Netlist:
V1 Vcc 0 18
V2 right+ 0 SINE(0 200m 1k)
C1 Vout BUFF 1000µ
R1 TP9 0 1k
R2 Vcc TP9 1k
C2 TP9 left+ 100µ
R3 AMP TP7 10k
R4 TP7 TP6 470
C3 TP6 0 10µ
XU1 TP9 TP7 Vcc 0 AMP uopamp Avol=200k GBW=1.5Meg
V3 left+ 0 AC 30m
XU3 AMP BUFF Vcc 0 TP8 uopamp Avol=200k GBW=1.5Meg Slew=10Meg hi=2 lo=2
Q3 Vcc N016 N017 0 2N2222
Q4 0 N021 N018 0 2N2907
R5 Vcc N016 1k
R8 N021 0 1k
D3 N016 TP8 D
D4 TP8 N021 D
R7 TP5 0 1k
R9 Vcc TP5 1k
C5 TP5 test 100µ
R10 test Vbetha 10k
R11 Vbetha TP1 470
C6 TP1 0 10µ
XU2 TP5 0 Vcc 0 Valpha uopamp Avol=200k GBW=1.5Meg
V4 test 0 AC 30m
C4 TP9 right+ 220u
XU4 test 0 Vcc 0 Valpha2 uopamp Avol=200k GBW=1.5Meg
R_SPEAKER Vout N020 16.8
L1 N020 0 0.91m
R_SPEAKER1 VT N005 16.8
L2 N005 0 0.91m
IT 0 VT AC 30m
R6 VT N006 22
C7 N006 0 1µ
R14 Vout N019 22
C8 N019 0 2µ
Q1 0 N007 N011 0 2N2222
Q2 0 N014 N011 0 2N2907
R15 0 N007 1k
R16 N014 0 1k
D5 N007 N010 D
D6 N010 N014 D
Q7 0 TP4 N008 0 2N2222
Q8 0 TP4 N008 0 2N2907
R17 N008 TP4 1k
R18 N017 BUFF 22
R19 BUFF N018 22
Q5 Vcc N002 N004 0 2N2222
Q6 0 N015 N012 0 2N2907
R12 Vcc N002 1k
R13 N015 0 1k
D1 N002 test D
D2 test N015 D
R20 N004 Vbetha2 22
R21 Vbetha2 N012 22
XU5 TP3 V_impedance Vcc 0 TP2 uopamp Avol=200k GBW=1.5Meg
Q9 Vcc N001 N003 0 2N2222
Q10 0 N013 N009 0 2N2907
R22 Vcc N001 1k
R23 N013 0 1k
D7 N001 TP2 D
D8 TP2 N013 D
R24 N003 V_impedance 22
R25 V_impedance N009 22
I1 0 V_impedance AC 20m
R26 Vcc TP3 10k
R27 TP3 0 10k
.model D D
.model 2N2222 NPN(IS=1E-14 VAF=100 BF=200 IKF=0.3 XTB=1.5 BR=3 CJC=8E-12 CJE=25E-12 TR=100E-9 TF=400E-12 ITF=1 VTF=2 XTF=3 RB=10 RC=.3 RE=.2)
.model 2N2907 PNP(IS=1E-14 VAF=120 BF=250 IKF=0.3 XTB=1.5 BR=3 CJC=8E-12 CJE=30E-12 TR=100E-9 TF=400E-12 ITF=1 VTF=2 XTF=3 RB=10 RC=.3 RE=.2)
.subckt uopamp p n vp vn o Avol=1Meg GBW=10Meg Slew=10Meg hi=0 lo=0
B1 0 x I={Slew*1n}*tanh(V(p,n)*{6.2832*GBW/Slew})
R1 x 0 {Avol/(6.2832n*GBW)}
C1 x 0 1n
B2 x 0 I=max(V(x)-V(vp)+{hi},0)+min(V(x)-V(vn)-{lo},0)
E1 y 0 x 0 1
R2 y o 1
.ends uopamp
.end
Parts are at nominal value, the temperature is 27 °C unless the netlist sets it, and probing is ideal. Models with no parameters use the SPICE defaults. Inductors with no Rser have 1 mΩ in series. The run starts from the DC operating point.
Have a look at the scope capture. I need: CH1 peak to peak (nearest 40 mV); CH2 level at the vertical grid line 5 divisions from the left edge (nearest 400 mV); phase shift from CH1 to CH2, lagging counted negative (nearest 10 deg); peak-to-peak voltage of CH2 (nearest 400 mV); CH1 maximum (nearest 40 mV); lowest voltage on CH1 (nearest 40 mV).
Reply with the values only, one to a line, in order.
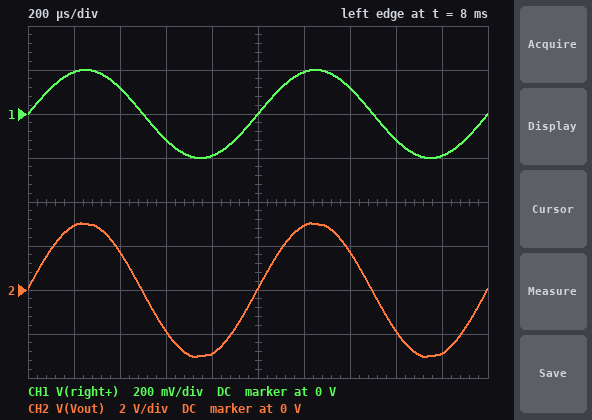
400 mV
0 V
0 deg
6.0 V
200 mV
-200 mV
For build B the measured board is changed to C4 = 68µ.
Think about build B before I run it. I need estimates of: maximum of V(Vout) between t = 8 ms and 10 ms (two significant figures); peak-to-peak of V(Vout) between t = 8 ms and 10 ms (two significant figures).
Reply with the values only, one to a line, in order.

1.8 V
3.6 V
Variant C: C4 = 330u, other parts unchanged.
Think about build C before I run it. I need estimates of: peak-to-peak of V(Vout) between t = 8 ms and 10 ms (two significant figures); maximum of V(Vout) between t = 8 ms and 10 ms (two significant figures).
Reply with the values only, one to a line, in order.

6.2 V
3.1 V
